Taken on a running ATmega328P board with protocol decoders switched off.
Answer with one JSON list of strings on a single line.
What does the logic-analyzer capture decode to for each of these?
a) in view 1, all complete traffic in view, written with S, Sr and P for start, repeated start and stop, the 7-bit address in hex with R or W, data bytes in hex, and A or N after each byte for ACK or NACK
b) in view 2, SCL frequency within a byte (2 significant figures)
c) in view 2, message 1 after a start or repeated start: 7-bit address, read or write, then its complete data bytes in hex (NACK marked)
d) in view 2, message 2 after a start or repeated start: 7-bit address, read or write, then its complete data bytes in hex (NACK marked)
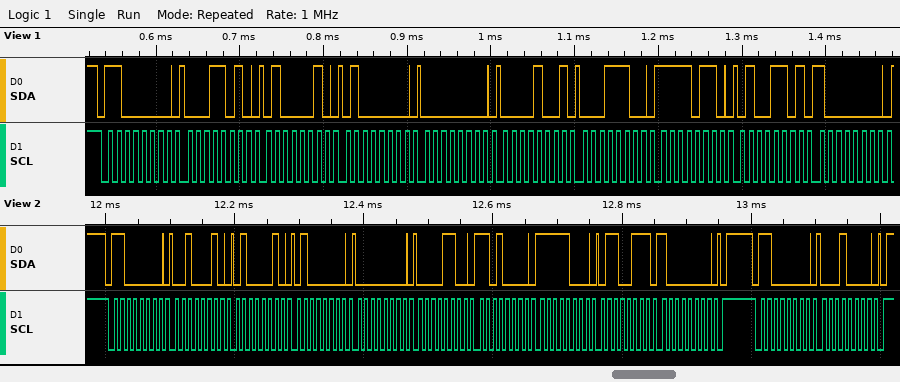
["S 60W A 1A A 42 A 40 A 00 A 09 A 1C A F6 A 4D A 80 A", "100 kHz", "0x60 write: 22 42 40 00 0C D0 F8 67 80", "0x60 write: 10"]
